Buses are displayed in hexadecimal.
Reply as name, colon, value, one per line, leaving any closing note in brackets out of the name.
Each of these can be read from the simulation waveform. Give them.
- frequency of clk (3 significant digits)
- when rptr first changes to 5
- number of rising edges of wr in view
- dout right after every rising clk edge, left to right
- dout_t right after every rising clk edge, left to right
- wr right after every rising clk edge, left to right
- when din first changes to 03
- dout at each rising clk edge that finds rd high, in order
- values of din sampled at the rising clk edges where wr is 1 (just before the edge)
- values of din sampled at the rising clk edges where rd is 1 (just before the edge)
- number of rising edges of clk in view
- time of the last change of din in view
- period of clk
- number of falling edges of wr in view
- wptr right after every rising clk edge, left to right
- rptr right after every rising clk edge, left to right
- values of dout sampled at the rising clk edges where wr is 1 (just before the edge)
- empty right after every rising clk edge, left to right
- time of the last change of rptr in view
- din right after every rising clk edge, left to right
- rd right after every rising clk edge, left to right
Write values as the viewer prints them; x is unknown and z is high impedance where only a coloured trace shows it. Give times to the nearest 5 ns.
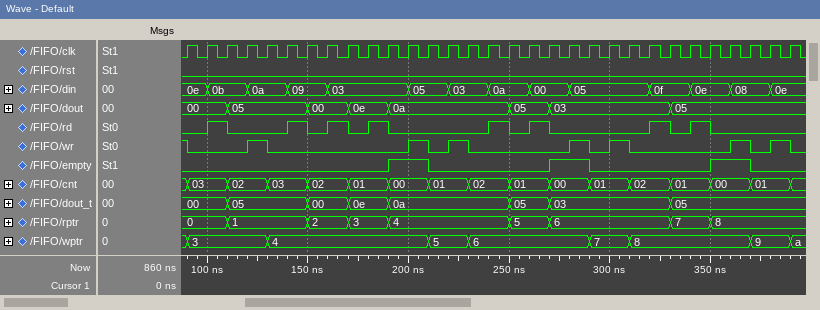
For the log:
frequency of clk: 100 MHz
when rptr first changes to 5: 250 ns
number of rising edges of wr in view: 7
dout right after every rising clk edge, left to right: 00, 00, 05, 05, 05, 05, 00, 00, 0e, 0e, 0a, 0a, 0a, 0a, 0a, 0a, 05, 05, 03, 03, 03, 03, 03, 03, 05, 05, 05, 05, 05, 05, 05
dout_t right after every rising clk edge, left to right: 00, 00, 05, 05, 05, 05, 00, 00, 0e, 0e, 0a, 0a, 0a, 0a, 0a, 0a, 05, 05, 03, 03, 03, 03, 03, 03, 05, 05, 05, 05, 05, 05, 05
wr right after every rising clk edge, left to right: 0 0 0 1 0 0 0 0 0 0 0 1 0 1 0 0 0 0 0 1 0 1 0 0 0 0 0 1 0 1 0
when din first changes to 03: 160 ns
dout at each rising clk edge that finds rd high, in order: 00, 05, 00, 0e, 0a, 05, 03, 05
values of din sampled at the rising clk edges where wr is 1: 0e, 0a, 05, 03, 05, 05, 08, 0e
values of din sampled at the rising clk edges where rd is 1: 0b, 09, 03, 03, 0a, 00, 0f, 0e
number of rising edges of clk in view: 31
time of the last change of din in view: 380 ns
period of clk: 10 ns
number of falling edges of wr in view: 8
wptr right after every rising clk edge, left to right: 3, 3, 3, 3, 4, 4, 4, 4, 4, 4, 4, 4, 5, 5, 6, 6, 6, 6, 6, 6, 7, 7, 8, 8, 8, 8, 8, 8, 9, 9, a
rptr right after every rising clk edge, left to right: 0, 0, 1, 1, 1, 1, 2, 2, 3, 3, 4, 4, 4, 4, 4, 4, 5, 5, 6, 6, 6, 6, 6, 6, 7, 7, 8, 8, 8, 8, 8
values of dout sampled at the rising clk edges where wr is 1: 00, 05, 0a, 0a, 03, 03, 05, 05
empty right after every rising clk edge, left to right: 0 0 0 0 0 0 0 0 0 0 1 1 0 0 0 0 0 0 1 1 0 0 0 0 0 0 1 1 0 0 0
time of the last change of rptr in view: 350 ns
din right after every rising clk edge, left to right: 0e, 0b, 0b, 0a, 0a, 09, 09, 03, 03, 03, 03, 05, 05, 03, 03, 0a, 0a, 00, 00, 05, 05, 05, 05, 0f, 0f, 0e, 0e, 08, 08, 0e, 0e
rd right after every rising clk edge, left to right: 0 1 0 0 0 1 0 1 0 1 0 0 0 0 0 1 0 1 0 0 0 0 0 1 0 1 0 0 0 0 0
